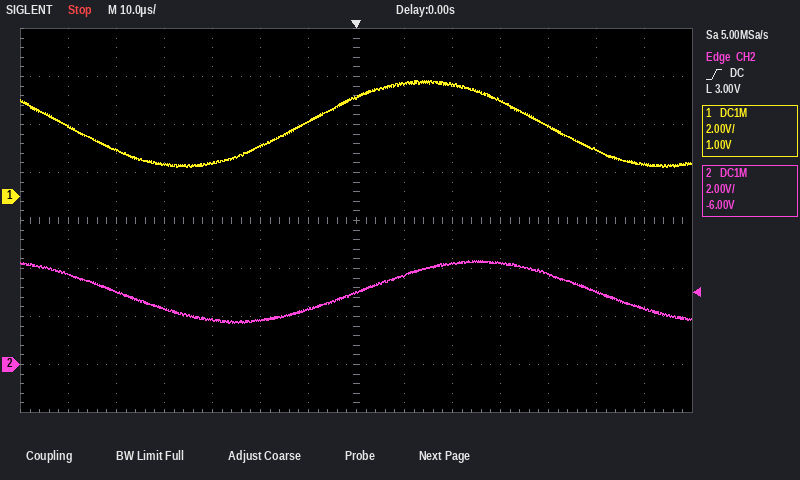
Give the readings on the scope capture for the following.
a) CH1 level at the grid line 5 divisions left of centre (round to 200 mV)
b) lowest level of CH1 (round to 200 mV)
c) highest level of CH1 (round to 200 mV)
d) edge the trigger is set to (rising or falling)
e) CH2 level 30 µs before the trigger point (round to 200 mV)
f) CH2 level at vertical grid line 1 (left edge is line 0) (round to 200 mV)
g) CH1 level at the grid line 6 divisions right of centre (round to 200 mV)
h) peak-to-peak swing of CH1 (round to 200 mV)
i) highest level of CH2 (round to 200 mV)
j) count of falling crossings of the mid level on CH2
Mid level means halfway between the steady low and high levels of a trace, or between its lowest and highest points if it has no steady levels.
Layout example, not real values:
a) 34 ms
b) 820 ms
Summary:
a) 2.0 V
b) 1.2 V
c) 4.8 V
d) rising
e) 1.8 V
f) 3.8 V
g) 1.4 V
h) 3.6 V
i) 4.4 V
j) 2
